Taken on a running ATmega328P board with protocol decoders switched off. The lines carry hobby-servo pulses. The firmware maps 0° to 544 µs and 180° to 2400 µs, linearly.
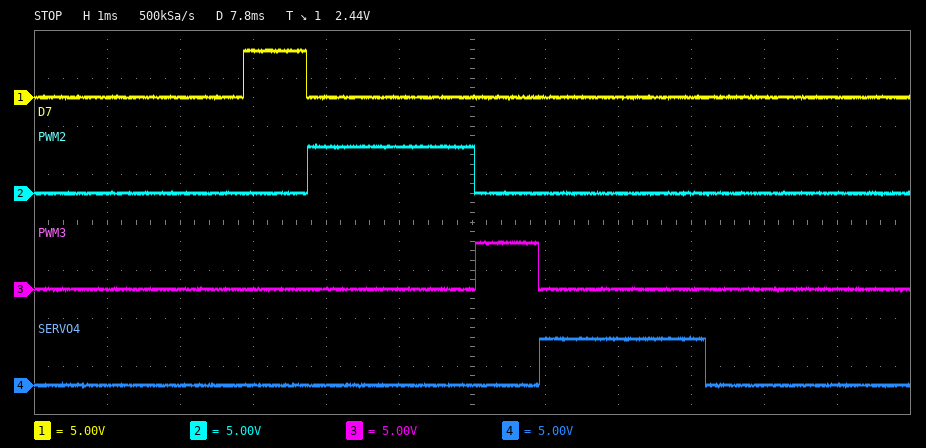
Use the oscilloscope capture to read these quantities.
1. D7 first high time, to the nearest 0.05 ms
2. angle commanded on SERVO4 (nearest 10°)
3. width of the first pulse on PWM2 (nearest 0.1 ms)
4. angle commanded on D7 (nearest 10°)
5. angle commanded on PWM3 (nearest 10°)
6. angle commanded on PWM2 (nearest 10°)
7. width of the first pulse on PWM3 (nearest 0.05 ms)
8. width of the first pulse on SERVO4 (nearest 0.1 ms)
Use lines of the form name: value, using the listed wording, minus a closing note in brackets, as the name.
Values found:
D7 first high time, to the nearest 0.05 ms: 0.85 ms
angle commanded on SERVO4: 170°
width of the first pulse on PWM2: 2.3 ms
angle commanded on D7: 30°
angle commanded on PWM3: 30°
angle commanded on PWM2: 170°
width of the first pulse on PWM3: 0.85 ms
width of the first pulse on SERVO4: 2.3 ms
